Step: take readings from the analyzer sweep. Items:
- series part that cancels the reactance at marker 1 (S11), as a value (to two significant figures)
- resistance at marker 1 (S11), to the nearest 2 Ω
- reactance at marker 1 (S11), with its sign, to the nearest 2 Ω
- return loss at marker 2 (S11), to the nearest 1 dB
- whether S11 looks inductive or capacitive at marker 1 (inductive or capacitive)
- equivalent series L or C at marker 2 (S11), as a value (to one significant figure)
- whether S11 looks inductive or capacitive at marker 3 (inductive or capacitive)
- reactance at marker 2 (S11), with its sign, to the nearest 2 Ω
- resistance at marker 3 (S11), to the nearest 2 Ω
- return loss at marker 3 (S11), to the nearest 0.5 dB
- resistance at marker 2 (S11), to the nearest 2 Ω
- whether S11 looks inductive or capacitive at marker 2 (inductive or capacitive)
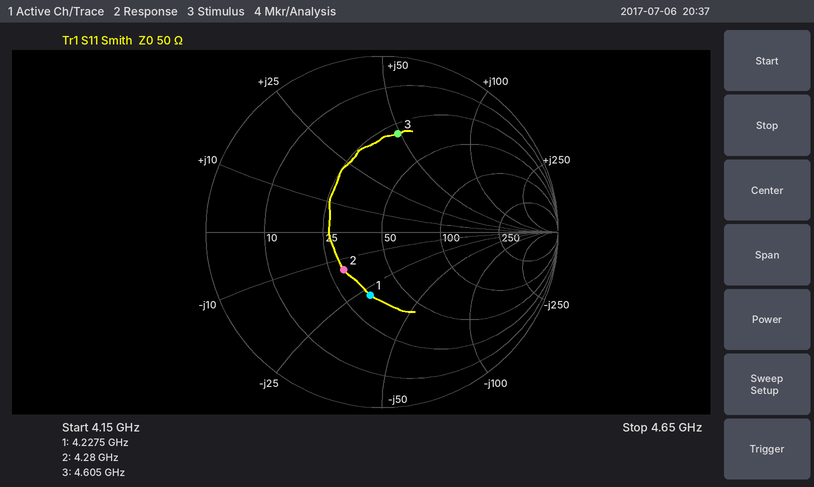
1.1 nH
34 Ω
-28 Ω
10 dB
capacitive
3 pF
inductive
-14 Ω
30 Ω
5.0 dB
30 Ω
capacitive
